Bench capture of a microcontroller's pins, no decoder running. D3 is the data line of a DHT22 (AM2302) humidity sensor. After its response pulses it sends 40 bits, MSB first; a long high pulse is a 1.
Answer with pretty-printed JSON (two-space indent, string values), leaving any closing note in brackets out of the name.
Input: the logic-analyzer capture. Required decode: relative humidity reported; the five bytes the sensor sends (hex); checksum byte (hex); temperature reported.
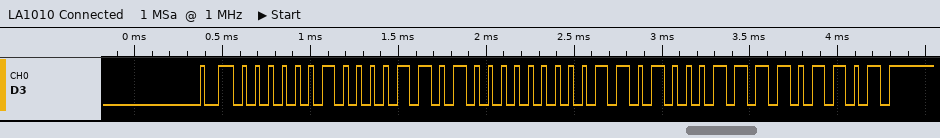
{
  "relative humidity reported": "53.8 %",
  "the five bytes the sensor sends": "02 1A 00 D1 ED",
  "checksum byte": "0xED",
  "temperature reported": "20.9 °C"
}
